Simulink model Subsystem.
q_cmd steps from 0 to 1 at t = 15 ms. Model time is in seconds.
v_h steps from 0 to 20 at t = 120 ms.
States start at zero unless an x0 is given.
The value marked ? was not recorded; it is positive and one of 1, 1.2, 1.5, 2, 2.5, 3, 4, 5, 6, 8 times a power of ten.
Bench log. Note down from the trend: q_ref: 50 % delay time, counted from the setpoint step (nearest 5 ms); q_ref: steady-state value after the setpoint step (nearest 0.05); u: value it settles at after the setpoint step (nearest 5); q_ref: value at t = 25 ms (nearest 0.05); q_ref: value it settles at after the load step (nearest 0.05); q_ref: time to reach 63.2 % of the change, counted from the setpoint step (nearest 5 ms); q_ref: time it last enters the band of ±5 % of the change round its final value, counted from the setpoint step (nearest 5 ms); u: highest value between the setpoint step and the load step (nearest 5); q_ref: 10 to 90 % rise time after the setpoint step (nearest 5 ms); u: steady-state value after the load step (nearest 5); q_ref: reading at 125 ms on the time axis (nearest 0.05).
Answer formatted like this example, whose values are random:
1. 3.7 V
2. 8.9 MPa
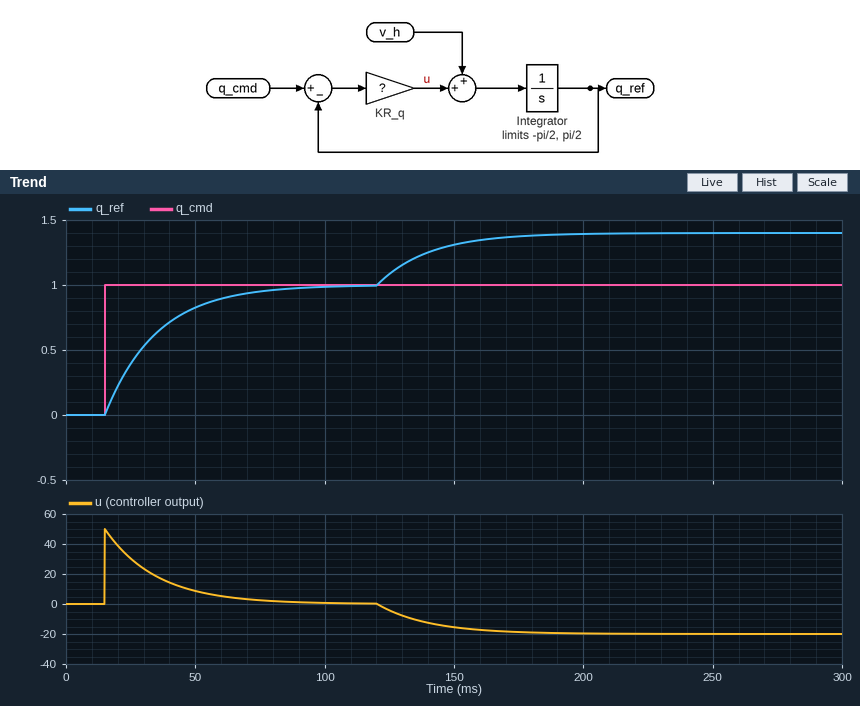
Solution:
1. 15 ms
2. 1.00
3. 0
4. 0.40
5. 1.40
6. 20 ms
7. 60 ms
8. 50
9. 45 ms
10. -20
11. 1.10
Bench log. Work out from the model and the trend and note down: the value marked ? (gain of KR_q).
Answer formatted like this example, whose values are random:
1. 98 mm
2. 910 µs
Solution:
1. 50
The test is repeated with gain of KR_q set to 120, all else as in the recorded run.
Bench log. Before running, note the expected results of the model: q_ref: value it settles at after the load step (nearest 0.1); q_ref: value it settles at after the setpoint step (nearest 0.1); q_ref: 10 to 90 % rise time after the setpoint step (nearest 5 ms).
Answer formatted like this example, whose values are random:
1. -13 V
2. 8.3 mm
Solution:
1. 1.2
2. 1.0
3. 20 ms
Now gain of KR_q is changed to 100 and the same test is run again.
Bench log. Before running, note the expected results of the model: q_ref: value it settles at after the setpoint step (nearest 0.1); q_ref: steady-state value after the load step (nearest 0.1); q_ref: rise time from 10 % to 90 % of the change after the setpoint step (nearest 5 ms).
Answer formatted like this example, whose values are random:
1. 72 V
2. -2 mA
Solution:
1. 1.0
2. 1.2
3. 20 ms
